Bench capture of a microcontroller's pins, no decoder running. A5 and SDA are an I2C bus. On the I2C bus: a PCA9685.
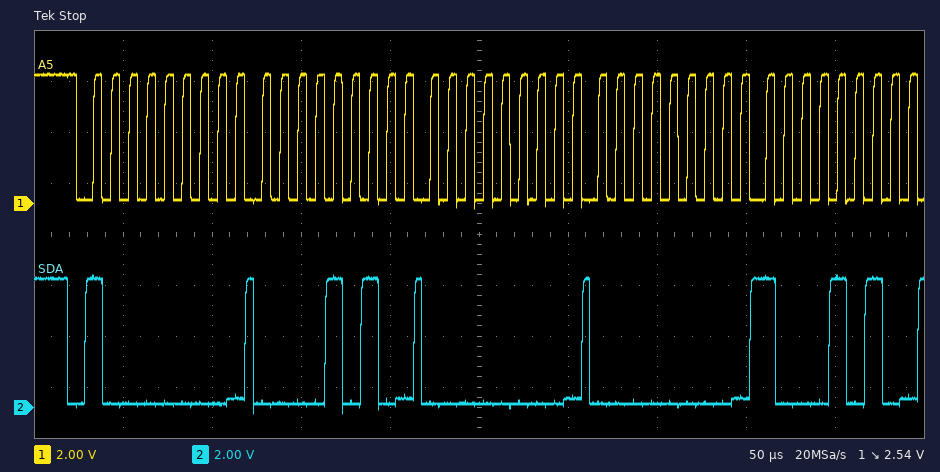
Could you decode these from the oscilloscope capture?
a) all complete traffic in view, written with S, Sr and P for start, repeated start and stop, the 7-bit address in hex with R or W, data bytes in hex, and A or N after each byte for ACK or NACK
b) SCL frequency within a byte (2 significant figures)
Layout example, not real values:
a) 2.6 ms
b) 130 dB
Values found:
a) S 40W A 0A A 00 A 00 A 8A A
b) 100 kHz
